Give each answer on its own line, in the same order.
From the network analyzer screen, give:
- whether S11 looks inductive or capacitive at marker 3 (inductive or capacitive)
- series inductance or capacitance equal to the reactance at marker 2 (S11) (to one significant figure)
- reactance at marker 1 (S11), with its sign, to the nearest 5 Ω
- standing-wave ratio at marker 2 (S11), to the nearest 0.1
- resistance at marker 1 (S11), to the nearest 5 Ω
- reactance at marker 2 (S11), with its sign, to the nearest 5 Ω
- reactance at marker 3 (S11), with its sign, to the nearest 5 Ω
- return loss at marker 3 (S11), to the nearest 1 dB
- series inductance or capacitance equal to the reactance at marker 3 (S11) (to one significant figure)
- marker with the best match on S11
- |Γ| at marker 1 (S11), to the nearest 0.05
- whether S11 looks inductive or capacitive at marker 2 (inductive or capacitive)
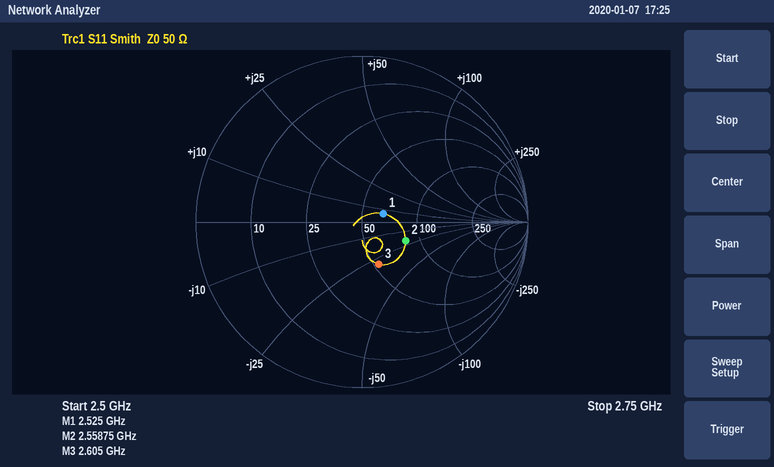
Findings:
capacitive
3 pF
+5 Ω
1.8
65 Ω
-20 Ω
-30 Ω
11 dB
2 pF
marker 1
0.15
capacitive
